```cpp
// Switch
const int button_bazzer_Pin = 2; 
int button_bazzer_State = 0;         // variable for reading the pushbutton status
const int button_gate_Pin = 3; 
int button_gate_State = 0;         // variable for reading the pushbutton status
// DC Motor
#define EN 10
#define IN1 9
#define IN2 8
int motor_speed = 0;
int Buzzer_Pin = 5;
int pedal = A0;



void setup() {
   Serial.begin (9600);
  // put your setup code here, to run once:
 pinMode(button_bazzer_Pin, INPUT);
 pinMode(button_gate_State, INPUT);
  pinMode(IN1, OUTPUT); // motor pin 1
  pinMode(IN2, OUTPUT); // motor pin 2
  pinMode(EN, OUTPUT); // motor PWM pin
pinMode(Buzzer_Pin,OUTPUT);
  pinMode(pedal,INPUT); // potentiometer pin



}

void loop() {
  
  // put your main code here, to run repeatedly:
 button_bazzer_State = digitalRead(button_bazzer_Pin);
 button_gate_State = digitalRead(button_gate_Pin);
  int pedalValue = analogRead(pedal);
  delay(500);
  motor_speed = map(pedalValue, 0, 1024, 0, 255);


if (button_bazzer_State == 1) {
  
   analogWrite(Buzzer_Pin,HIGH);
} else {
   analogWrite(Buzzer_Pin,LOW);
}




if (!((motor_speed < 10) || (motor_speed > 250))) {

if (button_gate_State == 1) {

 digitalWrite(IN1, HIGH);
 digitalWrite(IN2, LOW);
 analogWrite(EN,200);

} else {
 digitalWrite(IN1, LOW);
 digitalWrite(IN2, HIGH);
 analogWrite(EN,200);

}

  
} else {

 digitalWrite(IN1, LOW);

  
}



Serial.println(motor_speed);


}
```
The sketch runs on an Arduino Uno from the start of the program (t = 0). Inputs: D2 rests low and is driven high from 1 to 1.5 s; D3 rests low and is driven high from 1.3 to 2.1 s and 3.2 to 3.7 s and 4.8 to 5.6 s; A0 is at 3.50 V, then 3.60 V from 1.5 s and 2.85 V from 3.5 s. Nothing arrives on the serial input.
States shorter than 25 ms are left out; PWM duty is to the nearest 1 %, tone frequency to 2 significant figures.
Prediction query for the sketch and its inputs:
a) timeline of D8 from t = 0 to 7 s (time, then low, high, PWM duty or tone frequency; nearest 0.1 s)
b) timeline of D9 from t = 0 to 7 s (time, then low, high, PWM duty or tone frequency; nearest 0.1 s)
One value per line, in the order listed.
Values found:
0 s low; 0.5 s high; 2 s low; 3 s high; 4 s low; 4.5 s high; 5.5 s low; 6.5 s high
0 s low; 2 s high; 3 s low; 4 s high; 4.5 s low; 5.5 s high; 6.5 s low
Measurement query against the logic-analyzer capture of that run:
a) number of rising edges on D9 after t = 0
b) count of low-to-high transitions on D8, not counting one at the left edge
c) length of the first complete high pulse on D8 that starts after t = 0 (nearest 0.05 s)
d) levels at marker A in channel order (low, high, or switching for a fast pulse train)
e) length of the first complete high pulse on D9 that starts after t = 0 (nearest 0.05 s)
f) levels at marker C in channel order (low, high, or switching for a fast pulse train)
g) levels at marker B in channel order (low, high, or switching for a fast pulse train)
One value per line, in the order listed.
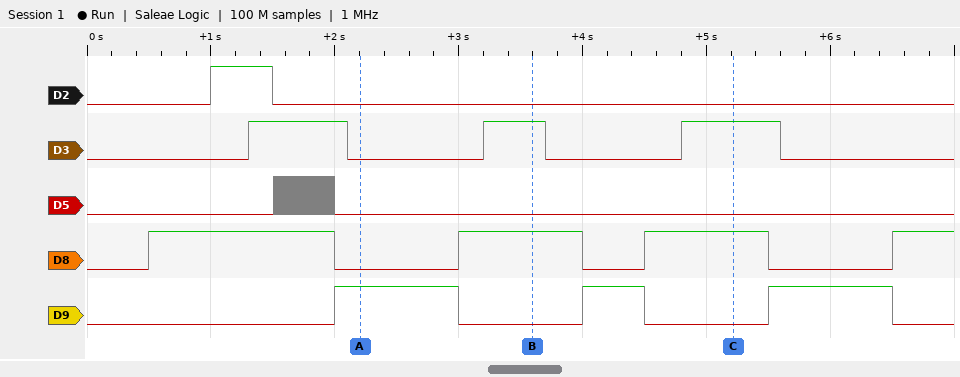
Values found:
3
4
1.50 s
D2 low, D3 low, D5 low, D8 low, D9 high
1.00 s
D2 low, D3 high, D5 low, D8 high, D9 low
D2 low, D3 high, D5 low, D8 high, D9 low
